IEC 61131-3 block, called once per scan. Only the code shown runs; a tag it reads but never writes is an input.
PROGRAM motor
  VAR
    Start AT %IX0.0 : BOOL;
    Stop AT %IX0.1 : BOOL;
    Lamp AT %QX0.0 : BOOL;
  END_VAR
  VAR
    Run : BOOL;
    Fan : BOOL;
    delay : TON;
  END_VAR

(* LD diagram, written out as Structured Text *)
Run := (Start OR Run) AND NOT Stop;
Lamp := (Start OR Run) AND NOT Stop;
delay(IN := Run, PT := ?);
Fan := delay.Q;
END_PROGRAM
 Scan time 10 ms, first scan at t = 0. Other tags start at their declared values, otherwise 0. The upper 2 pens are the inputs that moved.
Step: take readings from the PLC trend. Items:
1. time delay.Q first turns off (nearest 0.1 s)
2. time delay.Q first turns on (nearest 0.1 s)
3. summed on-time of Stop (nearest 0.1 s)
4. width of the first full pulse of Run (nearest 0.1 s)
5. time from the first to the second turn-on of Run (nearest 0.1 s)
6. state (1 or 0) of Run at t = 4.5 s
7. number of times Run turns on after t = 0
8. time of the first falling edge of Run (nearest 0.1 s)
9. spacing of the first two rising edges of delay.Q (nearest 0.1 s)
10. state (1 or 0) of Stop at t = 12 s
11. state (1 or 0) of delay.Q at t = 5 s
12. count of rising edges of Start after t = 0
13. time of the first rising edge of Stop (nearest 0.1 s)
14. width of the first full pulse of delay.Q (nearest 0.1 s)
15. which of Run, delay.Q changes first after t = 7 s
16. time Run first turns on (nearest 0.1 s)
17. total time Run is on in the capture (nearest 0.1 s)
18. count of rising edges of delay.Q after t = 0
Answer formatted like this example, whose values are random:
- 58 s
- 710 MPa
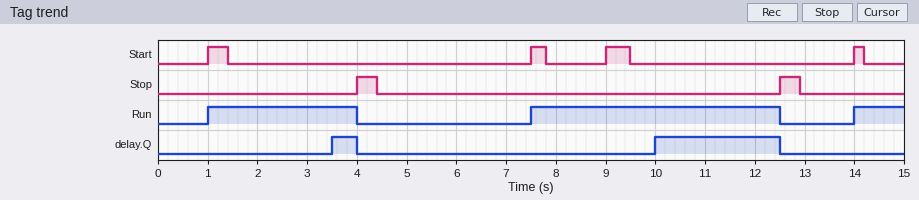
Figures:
- 4.0 s
- 3.5 s
- 0.8 s
- 3.0 s
- 6.5 s
- 0
- 3
- 4.0 s
- 6.5 s
- 0
- 0
- 4
- 4.0 s
- 0.5 s
- Run
- 1.0 s
- 9.0 s
- 2
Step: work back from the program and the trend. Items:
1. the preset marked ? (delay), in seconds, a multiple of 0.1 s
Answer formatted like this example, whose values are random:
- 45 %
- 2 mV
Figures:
- 2.5 s
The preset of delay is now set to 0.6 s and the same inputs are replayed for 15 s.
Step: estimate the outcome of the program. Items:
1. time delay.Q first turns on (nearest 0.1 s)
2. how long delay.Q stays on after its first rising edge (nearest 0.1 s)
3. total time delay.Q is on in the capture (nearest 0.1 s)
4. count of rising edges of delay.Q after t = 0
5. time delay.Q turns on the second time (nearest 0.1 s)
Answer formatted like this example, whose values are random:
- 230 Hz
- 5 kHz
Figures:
- 1.6 s
- 2.4 s
- 7.2 s
- 3
- 8.1 s
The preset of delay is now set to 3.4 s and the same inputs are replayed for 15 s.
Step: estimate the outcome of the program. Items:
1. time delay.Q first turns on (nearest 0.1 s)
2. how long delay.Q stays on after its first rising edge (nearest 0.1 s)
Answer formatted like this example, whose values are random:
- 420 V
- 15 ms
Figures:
- 10.9 s
- 1.6 s
